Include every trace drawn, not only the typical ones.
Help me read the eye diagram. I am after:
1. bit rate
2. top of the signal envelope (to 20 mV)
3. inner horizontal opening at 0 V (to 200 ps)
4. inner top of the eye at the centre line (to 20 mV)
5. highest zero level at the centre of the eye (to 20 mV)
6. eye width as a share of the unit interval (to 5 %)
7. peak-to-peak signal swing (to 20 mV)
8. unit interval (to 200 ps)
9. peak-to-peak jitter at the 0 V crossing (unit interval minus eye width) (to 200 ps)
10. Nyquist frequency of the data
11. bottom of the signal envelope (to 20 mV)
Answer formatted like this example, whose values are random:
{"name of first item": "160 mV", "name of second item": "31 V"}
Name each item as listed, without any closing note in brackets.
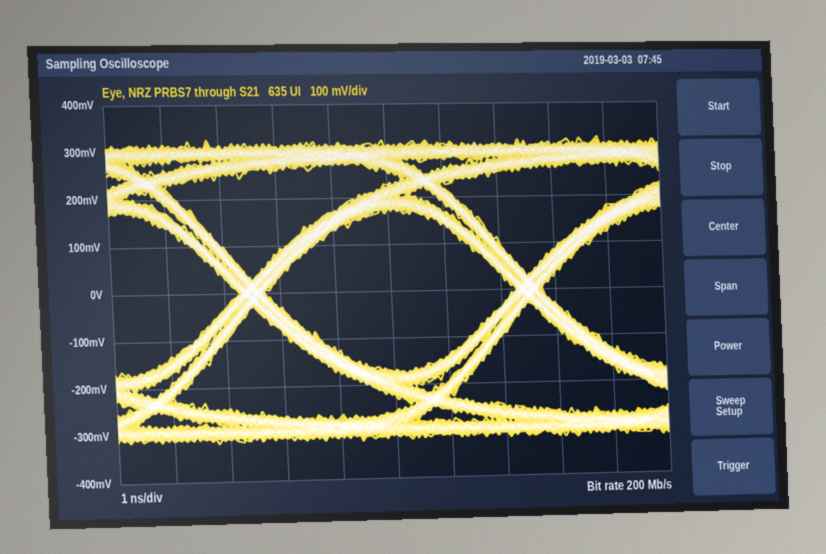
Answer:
{"bit rate": "200 Mb/s", "top of the signal envelope": "320 mV", "inner horizontal opening at 0 V": "4.6 ns", "inner top of the eye at the centre line": "180 mV", "highest zero level at the centre of the eye": "-180 mV", "eye width as a share of the unit interval": "90 %", "peak-to-peak signal swing": "640 mV", "unit interval": "5.0 ns", "peak-to-peak jitter at the 0 V crossing (unit interval minus eye width)": "400 ps", "Nyquist frequency of the data": "100 MHz", "bottom of the signal envelope": "-320 mV"}
